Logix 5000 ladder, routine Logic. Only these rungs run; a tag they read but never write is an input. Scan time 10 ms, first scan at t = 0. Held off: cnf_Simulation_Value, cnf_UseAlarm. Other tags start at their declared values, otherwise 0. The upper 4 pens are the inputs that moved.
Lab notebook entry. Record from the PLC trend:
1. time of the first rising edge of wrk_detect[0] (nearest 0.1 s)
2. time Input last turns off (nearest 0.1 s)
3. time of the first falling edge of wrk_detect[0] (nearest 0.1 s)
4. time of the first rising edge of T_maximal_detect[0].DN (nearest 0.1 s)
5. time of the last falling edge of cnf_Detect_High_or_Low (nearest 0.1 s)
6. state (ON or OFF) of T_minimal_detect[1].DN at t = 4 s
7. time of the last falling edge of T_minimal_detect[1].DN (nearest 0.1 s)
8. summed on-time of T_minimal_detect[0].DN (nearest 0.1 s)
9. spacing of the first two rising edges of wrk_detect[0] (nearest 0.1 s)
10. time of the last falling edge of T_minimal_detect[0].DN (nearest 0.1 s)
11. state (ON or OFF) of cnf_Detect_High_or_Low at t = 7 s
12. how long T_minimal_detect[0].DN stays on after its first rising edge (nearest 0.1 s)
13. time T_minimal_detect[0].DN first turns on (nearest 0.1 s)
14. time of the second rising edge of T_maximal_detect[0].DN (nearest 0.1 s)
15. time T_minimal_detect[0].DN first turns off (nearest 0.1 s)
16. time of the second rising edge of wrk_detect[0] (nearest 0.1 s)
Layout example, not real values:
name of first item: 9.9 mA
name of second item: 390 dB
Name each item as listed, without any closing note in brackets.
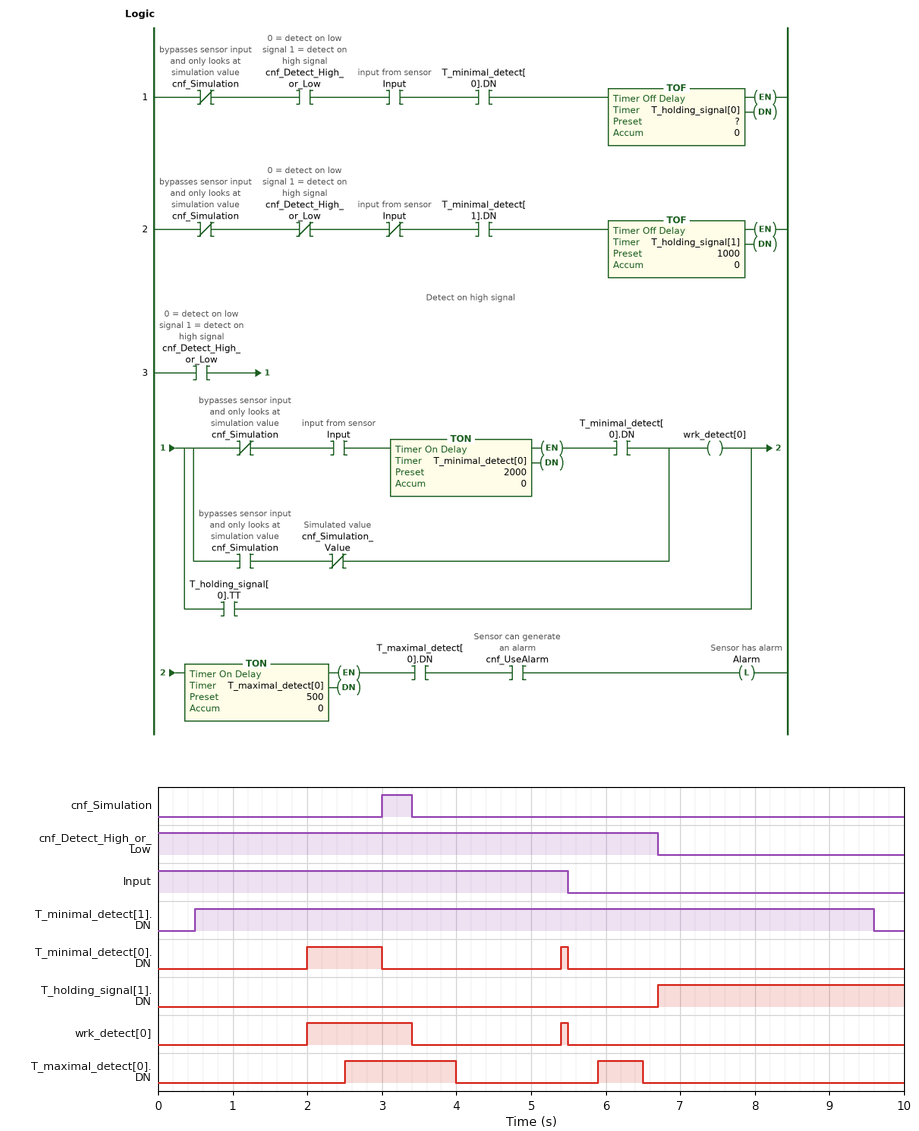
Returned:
time of the first rising edge of wrk_detect[0]: 2.0 s
time Input last turns off: 5.5 s
time of the first falling edge of wrk_detect[0]: 3.4 s
time of the first rising edge of T_maximal_detect[0].DN: 2.5 s
time of the last falling edge of cnf_Detect_High_or_Low: 6.7 s
state (ON or OFF) of T_minimal_detect[1].DN at t = 4 s: ON
time of the last falling edge of T_minimal_detect[1].DN: 9.6 s
summed on-time of T_minimal_detect[0].DN: 1.1 s
spacing of the first two rising edges of wrk_detect[0]: 3.4 s
time of the last falling edge of T_minimal_detect[0].DN: 5.5 s
state (ON or OFF) of cnf_Detect_High_or_Low at t = 7 s: OFF
how long T_minimal_detect[0].DN stays on after its first rising edge: 1.0 s
time T_minimal_detect[0].DN first turns on: 2.0 s
time of the second rising edge of T_maximal_detect[0].DN: 5.9 s
time T_minimal_detect[0].DN first turns off: 3.0 s
time of the second rising edge of wrk_detect[0]: 5.4 s
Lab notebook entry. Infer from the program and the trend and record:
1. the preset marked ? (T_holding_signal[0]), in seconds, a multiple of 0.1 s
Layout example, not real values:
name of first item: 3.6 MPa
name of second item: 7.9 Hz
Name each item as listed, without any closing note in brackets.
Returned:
the preset marked ? (T_holding_signal[0]), in seconds, a multiple of 0.1 s: 1.0 s
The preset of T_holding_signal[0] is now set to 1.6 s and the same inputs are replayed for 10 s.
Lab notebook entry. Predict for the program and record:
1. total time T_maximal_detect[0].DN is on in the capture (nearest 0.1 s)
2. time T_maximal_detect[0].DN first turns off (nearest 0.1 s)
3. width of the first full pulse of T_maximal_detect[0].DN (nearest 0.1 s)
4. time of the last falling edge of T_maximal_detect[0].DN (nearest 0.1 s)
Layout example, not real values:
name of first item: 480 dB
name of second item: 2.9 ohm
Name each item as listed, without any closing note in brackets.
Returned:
total time T_maximal_detect[0].DN is on in the capture: 2.9 s
time T_maximal_detect[0].DN first turns off: 4.6 s
width of the first full pulse of T_maximal_detect[0].DN: 2.1 s
time of the last falling edge of T_maximal_detect[0].DN: 6.7 s
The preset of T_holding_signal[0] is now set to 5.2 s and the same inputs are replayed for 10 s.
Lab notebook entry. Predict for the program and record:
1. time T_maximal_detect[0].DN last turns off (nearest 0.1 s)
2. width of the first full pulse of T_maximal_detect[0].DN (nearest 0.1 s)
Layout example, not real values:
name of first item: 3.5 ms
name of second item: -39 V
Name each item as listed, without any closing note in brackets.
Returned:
time T_maximal_detect[0].DN last turns off: 6.7 s
width of the first full pulse of T_maximal_detect[0].DN: 4.2 s
